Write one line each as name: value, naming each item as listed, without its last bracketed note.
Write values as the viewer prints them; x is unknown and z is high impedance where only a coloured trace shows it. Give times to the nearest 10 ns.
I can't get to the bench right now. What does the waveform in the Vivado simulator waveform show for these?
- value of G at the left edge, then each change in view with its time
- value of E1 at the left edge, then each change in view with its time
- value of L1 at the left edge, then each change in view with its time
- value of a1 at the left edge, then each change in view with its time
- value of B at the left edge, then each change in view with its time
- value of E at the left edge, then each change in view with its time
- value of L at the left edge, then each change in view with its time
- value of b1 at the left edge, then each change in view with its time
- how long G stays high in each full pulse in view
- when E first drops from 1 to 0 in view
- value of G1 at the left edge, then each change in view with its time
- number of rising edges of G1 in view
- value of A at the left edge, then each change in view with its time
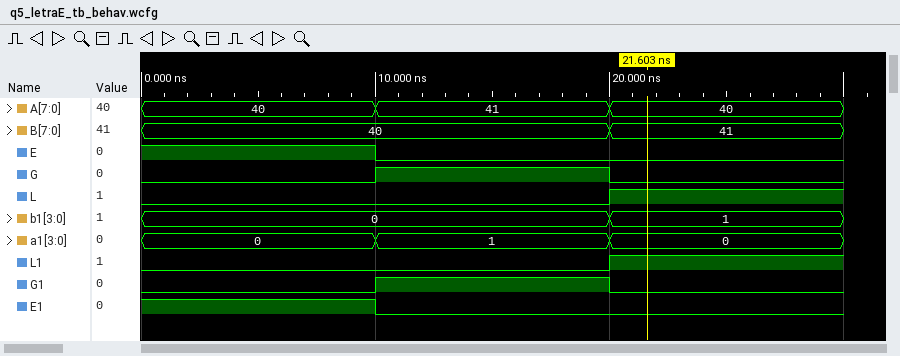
value of G at the left edge, then each change in view with its time: 0, 1 at 10 ns, 0 at 20 ns
value of E1 at the left edge, then each change in view with its time: 1, 0 at 10 ns
value of L1 at the left edge, then each change in view with its time: 0, 1 at 20 ns
value of a1 at the left edge, then each change in view with its time: 0, 1 at 10 ns, 0 at 20 ns
value of B at the left edge, then each change in view with its time: 40, 41 at 20 ns
value of E at the left edge, then each change in view with its time: 1, 0 at 10 ns
value of L at the left edge, then each change in view with its time: 0, 1 at 20 ns
value of b1 at the left edge, then each change in view with its time: 0, 1 at 20 ns
how long G stays high in each full pulse in view: 10 ns
when E first drops from 1 to 0 in view: 10 ns
value of G1 at the left edge, then each change in view with its time: 0, 1 at 10 ns, 0 at 20 ns
number of rising edges of G1 in view: 1
value of A at the left edge, then each change in view with its time: 40, 41 at 10 ns, 40 at 20 ns
